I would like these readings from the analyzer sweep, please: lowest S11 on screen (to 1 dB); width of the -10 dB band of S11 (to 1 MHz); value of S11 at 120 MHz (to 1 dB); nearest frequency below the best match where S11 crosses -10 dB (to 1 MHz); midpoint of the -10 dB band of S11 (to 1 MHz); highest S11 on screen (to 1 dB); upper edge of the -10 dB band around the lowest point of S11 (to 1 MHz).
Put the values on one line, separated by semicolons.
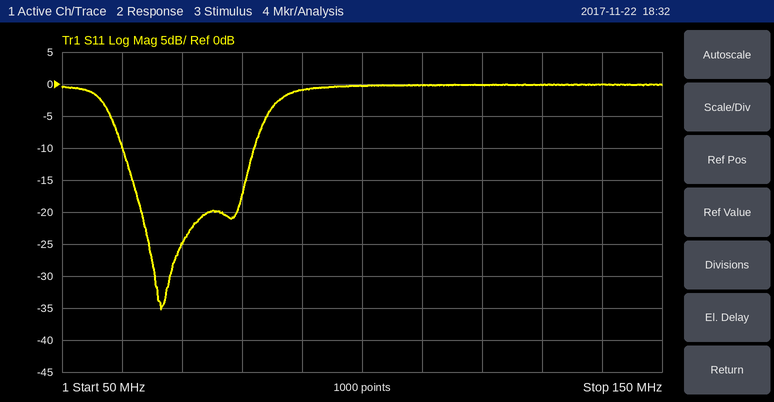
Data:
-35 dB; 22 MHz; 0 dB; 60 MHz; 71 MHz; 0 dB; 82 MHz
